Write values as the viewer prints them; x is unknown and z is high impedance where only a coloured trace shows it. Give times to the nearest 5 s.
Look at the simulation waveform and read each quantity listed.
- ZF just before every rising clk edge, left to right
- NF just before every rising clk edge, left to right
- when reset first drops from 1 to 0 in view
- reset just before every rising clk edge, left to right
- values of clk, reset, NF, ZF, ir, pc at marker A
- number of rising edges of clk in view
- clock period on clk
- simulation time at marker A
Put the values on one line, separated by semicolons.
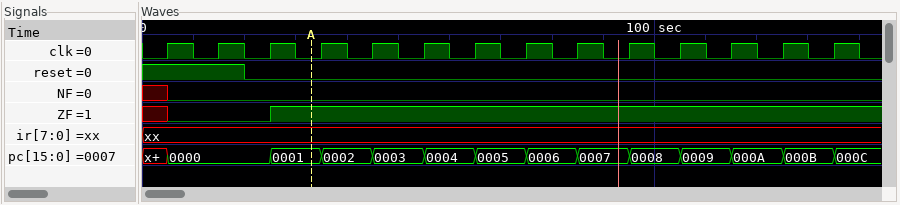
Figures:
x 0 0 1 1 1 1 1 1 1 1 1 1 1; x 0 0 0 0 0 0 0 0 0 0 0 0 0; 20 s; 1 1 0 0 0 0 0 0 0 0 0 0 0 0; clk=0, reset=0, NF=0, ZF=1, ir=xx, pc=0001; 14; 10 s; 35 s
